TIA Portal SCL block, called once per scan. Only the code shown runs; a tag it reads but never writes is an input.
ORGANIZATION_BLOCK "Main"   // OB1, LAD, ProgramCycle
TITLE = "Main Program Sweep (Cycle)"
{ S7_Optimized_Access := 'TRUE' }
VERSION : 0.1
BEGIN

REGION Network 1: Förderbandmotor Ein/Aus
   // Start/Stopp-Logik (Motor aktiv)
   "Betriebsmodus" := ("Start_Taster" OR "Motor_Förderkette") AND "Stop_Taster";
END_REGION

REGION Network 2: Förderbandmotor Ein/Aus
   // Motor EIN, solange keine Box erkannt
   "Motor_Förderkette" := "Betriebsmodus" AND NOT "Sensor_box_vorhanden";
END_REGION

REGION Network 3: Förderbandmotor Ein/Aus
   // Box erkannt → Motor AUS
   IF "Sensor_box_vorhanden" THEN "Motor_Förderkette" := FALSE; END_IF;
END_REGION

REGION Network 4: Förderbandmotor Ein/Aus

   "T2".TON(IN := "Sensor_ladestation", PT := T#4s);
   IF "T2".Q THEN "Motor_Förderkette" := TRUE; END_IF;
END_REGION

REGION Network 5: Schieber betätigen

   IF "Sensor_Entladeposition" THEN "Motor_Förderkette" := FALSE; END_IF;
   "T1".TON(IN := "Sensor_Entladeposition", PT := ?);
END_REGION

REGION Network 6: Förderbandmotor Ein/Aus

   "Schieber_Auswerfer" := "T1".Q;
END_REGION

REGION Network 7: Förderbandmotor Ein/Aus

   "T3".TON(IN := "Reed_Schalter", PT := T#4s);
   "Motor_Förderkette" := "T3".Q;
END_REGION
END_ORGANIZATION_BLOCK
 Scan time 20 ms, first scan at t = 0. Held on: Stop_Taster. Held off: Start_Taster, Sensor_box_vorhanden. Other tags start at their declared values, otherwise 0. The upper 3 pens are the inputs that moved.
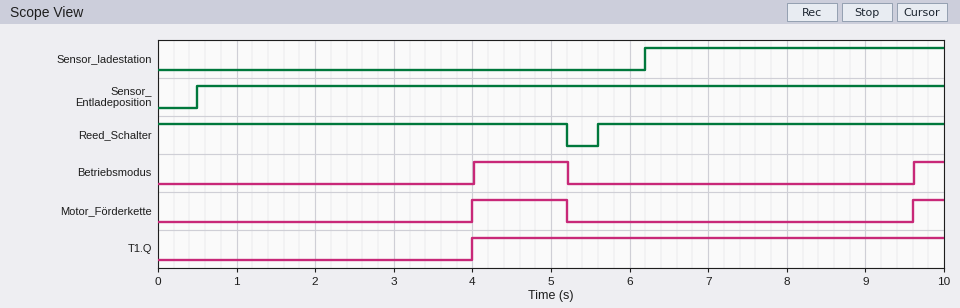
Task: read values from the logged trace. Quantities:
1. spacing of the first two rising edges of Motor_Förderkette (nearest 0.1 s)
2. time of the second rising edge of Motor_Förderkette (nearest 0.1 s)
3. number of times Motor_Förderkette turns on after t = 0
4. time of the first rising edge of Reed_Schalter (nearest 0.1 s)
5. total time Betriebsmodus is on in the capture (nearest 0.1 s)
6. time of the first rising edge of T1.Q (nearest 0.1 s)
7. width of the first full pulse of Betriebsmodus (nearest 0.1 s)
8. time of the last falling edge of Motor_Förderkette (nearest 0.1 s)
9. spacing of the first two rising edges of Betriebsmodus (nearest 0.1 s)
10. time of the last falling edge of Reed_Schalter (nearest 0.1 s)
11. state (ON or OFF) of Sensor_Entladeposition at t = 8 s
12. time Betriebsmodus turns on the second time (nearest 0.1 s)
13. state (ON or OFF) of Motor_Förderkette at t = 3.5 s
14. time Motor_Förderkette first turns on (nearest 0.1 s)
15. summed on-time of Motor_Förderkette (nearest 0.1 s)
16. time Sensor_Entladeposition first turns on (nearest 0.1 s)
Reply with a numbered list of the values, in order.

1. 5.6 s
2. 9.6 s
3. 2
4. 5.6 s
5. 1.6 s
6. 4.0 s
7. 1.2 s
8. 5.2 s
9. 5.6 s
10. 5.2 s
11. ON
12. 9.6 s
13. OFF
14. 4.0 s
15. 1.6 s
16. 0.5 s
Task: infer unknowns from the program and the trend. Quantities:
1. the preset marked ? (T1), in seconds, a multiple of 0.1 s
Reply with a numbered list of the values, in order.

1. 3.5 s
